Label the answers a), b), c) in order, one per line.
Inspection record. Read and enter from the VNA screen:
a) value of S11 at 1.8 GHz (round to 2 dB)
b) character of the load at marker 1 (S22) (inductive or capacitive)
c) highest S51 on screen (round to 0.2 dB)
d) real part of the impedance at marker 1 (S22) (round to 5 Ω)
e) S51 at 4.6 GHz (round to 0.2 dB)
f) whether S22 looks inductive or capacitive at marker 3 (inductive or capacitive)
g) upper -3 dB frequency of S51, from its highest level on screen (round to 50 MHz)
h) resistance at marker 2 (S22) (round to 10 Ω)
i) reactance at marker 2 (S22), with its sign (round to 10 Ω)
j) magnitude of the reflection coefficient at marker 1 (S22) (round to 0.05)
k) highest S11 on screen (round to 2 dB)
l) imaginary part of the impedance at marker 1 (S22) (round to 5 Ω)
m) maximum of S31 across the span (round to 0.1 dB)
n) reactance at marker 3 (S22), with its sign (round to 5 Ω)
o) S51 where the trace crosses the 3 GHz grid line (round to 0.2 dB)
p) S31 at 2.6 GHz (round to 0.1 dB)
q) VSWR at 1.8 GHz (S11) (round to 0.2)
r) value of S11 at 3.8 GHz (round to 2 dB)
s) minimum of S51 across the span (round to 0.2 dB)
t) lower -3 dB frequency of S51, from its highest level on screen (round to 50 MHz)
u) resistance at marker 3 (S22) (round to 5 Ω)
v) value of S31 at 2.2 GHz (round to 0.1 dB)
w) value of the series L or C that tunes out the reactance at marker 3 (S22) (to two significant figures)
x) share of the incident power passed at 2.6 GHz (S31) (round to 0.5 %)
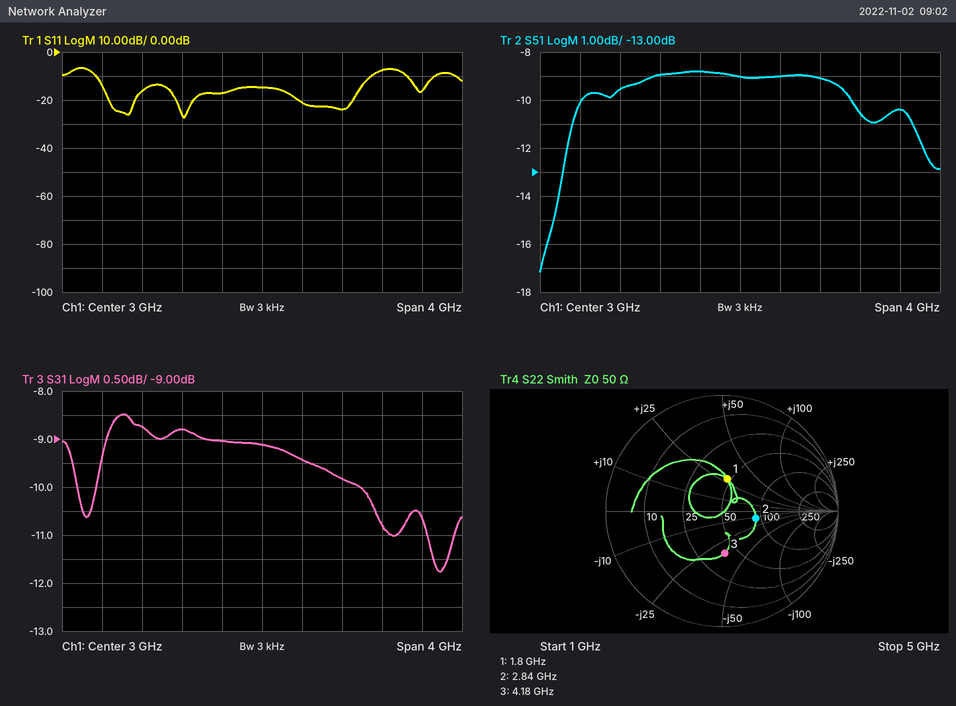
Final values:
a) -16 dB
b) inductive
c) -8.8 dB
d) 45 Ω
e) -10.4 dB
f) capacitive
g) 4.80 GHz
h) 90 Ω
i) -10 Ω
j) 0.30
k) -6 dB
l) +30 Ω
m) -8.5 dB
n) -35 Ω
o) -9.0 dB
p) -9.0 dB
q) 1.4
r) -24 dB
s) -17.2 dB
t) 1.30 GHz
u) 40 Ω
v) -8.8 dB
w) 1.3 nH
x) 12.5 %
